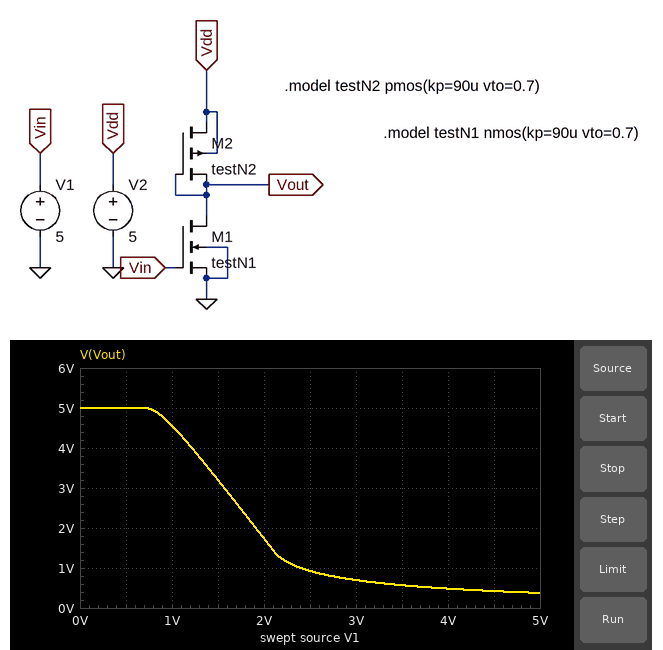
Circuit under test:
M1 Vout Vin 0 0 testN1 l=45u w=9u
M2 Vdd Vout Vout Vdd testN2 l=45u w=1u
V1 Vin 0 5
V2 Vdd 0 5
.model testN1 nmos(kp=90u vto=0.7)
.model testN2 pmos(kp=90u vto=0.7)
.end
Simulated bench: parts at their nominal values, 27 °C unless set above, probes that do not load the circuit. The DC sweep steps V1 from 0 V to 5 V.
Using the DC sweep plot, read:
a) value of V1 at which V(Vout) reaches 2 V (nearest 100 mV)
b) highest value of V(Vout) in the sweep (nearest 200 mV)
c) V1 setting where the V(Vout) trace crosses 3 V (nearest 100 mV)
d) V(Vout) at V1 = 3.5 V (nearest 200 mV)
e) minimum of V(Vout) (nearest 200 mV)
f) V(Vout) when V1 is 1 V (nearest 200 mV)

1.9 V
5.0 V
1.6 V
600 mV
400 mV
4.6 V
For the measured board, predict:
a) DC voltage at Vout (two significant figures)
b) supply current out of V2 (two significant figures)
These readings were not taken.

380 mV
28 µA
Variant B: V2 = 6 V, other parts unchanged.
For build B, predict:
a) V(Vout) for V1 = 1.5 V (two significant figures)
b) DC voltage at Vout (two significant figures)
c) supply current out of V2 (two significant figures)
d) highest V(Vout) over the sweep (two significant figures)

4.2 V
520 mV
38 µA
6.0 V
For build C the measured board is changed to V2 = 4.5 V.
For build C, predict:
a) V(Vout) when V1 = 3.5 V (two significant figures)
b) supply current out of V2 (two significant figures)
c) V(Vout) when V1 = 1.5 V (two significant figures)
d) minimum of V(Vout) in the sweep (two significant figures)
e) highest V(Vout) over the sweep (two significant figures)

470 mV
23 µA
2.7 V
310 mV
4.5 V
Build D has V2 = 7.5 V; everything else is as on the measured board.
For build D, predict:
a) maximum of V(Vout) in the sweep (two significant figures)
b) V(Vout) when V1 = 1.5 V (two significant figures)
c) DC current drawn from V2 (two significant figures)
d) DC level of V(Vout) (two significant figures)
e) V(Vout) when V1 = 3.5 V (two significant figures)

7.5 V
5.7 V
55 µA
780 mV
1.2 V
